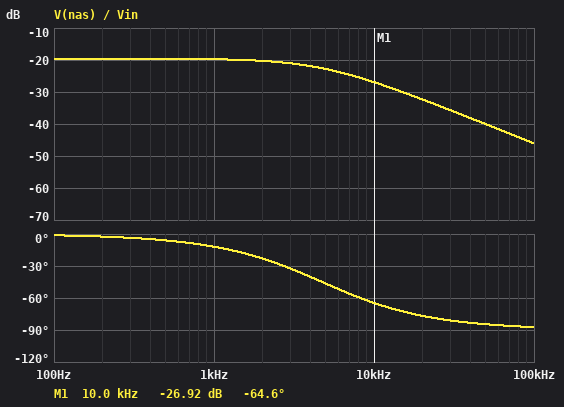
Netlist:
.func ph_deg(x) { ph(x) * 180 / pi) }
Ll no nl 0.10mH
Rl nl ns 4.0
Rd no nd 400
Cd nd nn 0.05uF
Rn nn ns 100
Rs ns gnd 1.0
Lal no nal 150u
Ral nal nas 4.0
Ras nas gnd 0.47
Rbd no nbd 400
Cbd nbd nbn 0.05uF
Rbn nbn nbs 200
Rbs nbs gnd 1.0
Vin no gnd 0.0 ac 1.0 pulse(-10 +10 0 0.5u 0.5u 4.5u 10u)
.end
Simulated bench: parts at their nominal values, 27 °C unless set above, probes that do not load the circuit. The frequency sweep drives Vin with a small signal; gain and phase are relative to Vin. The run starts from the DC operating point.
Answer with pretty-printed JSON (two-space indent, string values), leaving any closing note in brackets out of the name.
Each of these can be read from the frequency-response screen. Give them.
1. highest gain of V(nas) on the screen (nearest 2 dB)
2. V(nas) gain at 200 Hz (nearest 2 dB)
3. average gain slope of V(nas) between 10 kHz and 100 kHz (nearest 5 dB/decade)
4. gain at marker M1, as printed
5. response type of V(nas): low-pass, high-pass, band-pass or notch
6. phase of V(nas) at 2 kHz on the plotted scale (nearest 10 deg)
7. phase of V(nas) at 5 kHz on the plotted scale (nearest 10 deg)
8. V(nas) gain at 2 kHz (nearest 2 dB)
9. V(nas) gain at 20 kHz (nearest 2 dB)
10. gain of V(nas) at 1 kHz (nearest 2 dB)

{
  "highest gain of V(nas) on the screen": "-20 dB",
  "V(nas) gain at 200 Hz": "-20 dB",
  "average gain slope of V(nas) between 10 kHz and 100 kHz": "-20 dB/decade",
  "gain at marker M1, as printed": "-26.92 dB",
  "response type of V(nas): low-pass, high-pass, band-pass or notch": "low-pass",
  "phase of V(nas) at 2 kHz on the plotted scale": "-20 deg",
  "phase of V(nas) at 5 kHz on the plotted scale": "-50 deg",
  "V(nas) gain at 2 kHz": "-20 dB",
  "V(nas) gain at 20 kHz": "-32 dB",
  "gain of V(nas) at 1 kHz": "-20 dB"
}
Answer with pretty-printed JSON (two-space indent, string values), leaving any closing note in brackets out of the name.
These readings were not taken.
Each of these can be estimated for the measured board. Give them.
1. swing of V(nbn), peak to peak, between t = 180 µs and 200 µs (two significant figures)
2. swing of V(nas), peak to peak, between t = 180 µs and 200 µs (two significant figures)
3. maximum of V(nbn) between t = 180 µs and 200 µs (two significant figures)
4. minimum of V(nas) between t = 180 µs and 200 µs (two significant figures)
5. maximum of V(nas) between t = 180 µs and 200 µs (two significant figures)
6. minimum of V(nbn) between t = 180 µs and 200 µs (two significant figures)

{
  "swing of V(nbn), peak to peak, between t = 180 µs and 200 µs": "7.2 V",
  "swing of V(nas), peak to peak, between t = 180 µs and 200 µs": "150 mV",
  "maximum of V(nbn) between t = 180 µs and 200 µs": "3.6 V",
  "minimum of V(nas) between t = 180 µs and 200 µs": "-79 mV",
  "maximum of V(nas) between t = 180 µs and 200 µs": "71 mV",
  "minimum of V(nbn) between t = 180 µs and 200 µs": "-3.6 V"
}
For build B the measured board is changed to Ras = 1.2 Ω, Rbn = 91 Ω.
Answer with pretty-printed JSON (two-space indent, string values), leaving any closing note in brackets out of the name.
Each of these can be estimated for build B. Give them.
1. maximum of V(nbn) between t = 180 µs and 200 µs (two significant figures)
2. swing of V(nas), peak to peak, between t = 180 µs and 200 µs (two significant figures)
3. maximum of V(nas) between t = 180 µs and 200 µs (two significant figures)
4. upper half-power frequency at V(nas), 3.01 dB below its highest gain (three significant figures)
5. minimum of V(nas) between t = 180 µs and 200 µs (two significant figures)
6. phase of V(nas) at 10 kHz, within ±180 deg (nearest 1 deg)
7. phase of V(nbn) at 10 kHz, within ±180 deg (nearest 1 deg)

{
  "maximum of V(nbn) between t = 180 µs and 200 µs": "2.0 V",
  "swing of V(nas), peak to peak, between t = 180 µs and 200 µs": "380 mV",
  "maximum of V(nas) between t = 180 µs and 200 µs": "190 mV",
  "upper half-power frequency at V(nas), 3.01 dB below its highest gain": "5.52 kHz",
  "minimum of V(nas) between t = 180 µs and 200 µs": "-190 mV",
  "phase of V(nas) at 10 kHz, within ±180 deg": "-61 deg",
  "phase of V(nbn) at 10 kHz, within ±180 deg": "33 deg"
}
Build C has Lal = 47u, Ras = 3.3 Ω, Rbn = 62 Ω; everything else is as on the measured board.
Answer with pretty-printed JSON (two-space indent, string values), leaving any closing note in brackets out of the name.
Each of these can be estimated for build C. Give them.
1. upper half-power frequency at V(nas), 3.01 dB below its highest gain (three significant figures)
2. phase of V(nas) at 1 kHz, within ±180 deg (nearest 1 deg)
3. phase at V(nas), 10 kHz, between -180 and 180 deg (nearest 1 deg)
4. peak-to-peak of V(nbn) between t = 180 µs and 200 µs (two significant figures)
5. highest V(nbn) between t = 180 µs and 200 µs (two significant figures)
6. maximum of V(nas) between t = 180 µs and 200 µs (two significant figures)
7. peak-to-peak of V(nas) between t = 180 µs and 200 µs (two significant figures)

{
  "upper half-power frequency at V(nas), 3.01 dB below its highest gain": "24.7 kHz",
  "phase of V(nas) at 1 kHz, within ±180 deg": "-2 deg",
  "phase at V(nas), 10 kHz, between -180 and 180 deg": "-22 deg",
  "peak-to-peak of V(nbn) between t = 180 µs and 200 µs": "3.0 V",
  "highest V(nbn) between t = 180 µs and 200 µs": "1.5 V",
  "maximum of V(nas) between t = 180 µs and 200 µs": "1.6 V",
  "peak-to-peak of V(nas) between t = 180 µs and 200 µs": "3.2 V"
}
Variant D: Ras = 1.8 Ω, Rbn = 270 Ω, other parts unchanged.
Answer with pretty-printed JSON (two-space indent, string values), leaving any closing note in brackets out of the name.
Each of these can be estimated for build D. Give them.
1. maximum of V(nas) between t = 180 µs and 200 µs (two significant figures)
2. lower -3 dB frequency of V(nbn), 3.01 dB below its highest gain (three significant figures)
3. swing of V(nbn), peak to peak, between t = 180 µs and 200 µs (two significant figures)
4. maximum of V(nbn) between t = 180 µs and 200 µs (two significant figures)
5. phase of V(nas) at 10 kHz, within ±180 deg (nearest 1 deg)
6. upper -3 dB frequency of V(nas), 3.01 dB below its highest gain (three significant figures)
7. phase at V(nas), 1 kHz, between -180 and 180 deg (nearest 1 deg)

{
  "maximum of V(nas) between t = 180 µs and 200 µs": "280 mV",
  "lower -3 dB frequency of V(nbn), 3.01 dB below its highest gain": "4.74 kHz",
  "swing of V(nbn), peak to peak, between t = 180 µs and 200 µs": "8.6 V",
  "maximum of V(nbn) between t = 180 µs and 200 µs": "4.3 V",
  "phase of V(nas) at 10 kHz, within ±180 deg": "-58 deg",
  "upper -3 dB frequency of V(nas), 3.01 dB below its highest gain": "6.15 kHz",
  "phase at V(nas), 1 kHz, between -180 and 180 deg": "-9 deg"
}
